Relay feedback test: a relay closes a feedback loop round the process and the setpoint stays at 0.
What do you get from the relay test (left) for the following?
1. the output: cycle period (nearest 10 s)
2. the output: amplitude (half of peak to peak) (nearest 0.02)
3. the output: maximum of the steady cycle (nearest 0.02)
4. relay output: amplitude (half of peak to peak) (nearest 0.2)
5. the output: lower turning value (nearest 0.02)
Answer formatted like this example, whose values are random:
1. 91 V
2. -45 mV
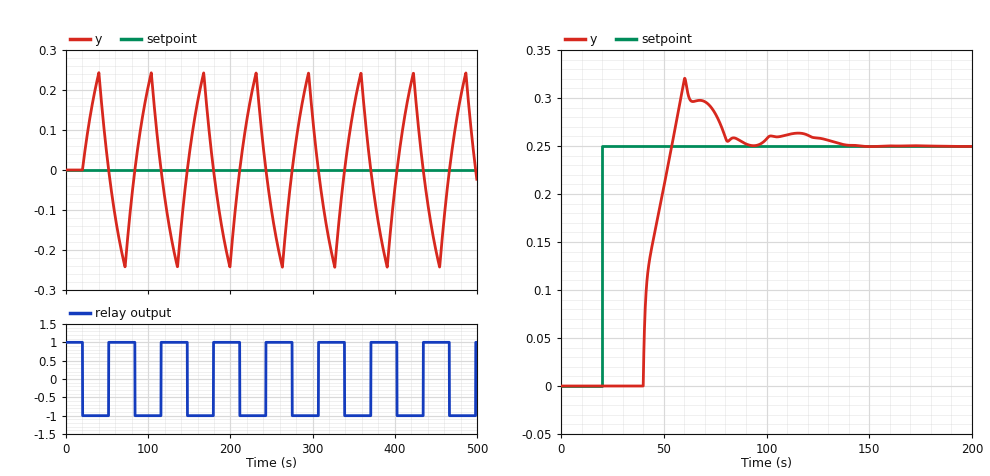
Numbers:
1. 60 s
2. 0.24
3. 0.24
4. 1.0
5. -0.24
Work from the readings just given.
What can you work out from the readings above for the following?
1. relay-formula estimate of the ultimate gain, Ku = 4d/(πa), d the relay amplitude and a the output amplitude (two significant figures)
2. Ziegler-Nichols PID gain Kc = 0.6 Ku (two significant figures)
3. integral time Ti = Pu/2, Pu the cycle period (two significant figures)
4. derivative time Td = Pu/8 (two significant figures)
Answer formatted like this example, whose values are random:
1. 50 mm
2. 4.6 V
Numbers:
1. 5.3
2. 3.2
3. 30 s
4. 7.5 s
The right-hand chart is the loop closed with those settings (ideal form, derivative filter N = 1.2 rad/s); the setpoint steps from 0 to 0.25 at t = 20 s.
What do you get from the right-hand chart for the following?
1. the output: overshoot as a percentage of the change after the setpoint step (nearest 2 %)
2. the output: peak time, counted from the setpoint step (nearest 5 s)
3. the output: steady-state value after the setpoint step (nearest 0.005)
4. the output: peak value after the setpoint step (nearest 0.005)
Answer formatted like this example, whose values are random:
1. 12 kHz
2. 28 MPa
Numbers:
1. 28 %
2. 40 s
3. 0.250
4. 0.320
